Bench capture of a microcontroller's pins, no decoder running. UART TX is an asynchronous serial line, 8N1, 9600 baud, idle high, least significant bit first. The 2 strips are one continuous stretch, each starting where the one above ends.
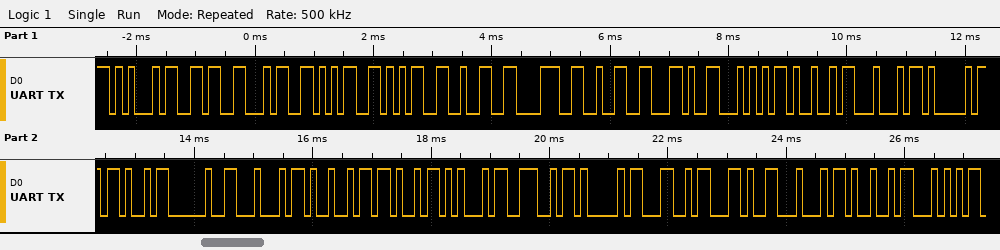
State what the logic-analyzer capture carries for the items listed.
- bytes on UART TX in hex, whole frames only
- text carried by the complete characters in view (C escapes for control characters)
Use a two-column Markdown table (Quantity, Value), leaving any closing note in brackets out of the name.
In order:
| Quantity | Value |
|---|---|
| bytes on UART TX in hex, whole frames only | 45 36 34 35 35 32 38 32 2C 54 49 44 41 4B 20 44 49 4B 45 4E 41 4C 2C 44 49 54 |
| text carried by the complete characters in view | "E6455282,TIDAK DIKENAL,DIT" |
